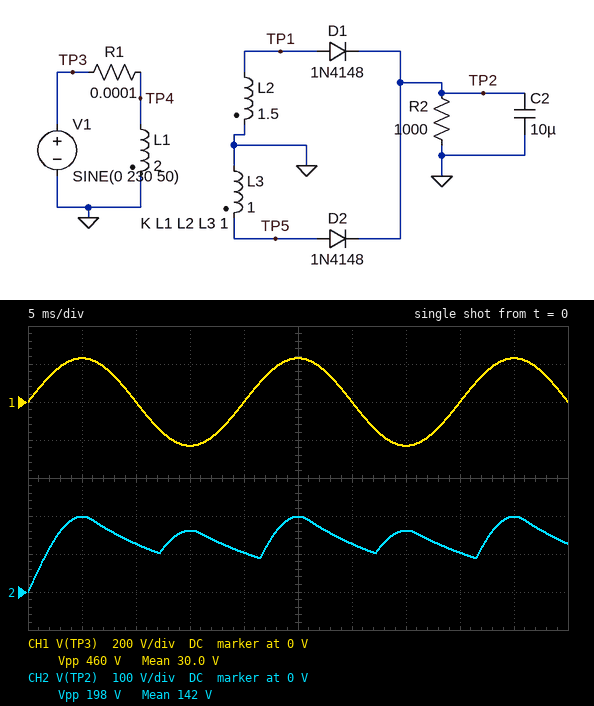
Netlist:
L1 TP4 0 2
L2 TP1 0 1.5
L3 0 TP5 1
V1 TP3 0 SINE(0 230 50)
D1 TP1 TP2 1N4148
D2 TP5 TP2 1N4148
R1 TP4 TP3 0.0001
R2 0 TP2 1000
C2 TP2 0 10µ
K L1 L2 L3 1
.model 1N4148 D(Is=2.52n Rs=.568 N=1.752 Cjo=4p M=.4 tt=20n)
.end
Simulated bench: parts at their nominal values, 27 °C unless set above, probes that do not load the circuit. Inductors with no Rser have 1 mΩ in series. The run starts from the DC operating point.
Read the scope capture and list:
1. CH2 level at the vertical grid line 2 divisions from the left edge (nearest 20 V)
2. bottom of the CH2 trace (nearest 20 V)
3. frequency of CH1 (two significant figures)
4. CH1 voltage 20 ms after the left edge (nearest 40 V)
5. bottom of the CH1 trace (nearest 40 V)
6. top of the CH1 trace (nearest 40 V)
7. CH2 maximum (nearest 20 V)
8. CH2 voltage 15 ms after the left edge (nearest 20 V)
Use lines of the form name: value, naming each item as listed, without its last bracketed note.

CH2 level at the vertical grid line 2 divisions from the left edge: 120 V
bottom of the CH2 trace: 0 V
frequency of CH1: 50 Hz
CH1 voltage 20 ms after the left edge: 0 V
bottom of the CH1 trace: -240 V
top of the CH1 trace: 240 V
CH2 maximum: 200 V
CH2 voltage 15 ms after the left edge: 160 V
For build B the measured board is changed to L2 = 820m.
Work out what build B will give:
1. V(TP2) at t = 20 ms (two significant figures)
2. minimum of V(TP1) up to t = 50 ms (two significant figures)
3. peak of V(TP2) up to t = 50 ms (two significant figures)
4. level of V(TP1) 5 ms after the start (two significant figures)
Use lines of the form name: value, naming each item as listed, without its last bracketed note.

V(TP2) at t = 20 ms: 100 V
minimum of V(TP1) up to t = 50 ms: -150 V
peak of V(TP2) up to t = 50 ms: 160 V
level of V(TP1) 5 ms after the start: 150 V
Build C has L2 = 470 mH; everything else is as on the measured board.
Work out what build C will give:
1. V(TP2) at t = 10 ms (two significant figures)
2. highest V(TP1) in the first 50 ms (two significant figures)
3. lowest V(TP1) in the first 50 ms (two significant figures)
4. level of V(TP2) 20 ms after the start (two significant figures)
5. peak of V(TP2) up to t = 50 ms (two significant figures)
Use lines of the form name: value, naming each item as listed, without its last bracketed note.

V(TP2) at t = 10 ms: 71 V
highest V(TP1) in the first 50 ms: 110 V
lowest V(TP1) in the first 50 ms: -110 V
level of V(TP2) 20 ms after the start: 100 V
peak of V(TP2) up to t = 50 ms: 160 V
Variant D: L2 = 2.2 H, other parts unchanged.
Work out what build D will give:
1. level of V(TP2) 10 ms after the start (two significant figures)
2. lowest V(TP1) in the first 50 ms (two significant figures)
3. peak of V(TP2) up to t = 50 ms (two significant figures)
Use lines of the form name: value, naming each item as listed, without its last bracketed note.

level of V(TP2) 10 ms after the start: 150 V
lowest V(TP1) in the first 50 ms: -240 V
peak of V(TP2) up to t = 50 ms: 240 V
